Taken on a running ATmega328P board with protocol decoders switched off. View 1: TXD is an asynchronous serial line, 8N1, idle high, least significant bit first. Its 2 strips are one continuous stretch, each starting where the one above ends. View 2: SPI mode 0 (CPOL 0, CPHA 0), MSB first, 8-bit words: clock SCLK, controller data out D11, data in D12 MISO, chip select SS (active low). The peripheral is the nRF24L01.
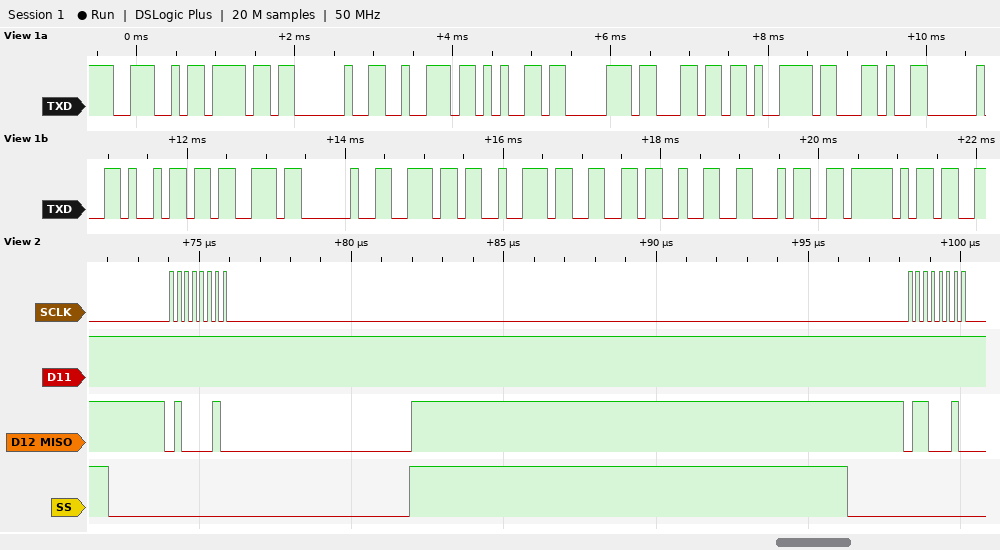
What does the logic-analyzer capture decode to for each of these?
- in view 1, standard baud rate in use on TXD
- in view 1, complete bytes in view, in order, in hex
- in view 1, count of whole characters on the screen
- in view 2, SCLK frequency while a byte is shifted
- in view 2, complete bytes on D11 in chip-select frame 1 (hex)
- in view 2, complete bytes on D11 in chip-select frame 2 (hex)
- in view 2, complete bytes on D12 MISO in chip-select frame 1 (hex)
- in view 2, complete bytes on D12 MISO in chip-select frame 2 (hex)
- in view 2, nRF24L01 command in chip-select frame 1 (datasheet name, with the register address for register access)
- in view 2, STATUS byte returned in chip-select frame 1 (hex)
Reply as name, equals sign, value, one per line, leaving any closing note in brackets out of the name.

in view 1, standard baud rate in use on TXD = 9600 baud
in view 1, complete bytes in view, in order, in hex = 0x4E 0x6F 0x20 0x72 0x65 0x70 0x6C 0x79 0x2C 0x20 0x69 0x73 0x20 0x6E 0x72 0x66 0x32 0x34 0x5F
in view 1, count of whole characters on the screen = 19
in view 2, SCLK frequency while a byte is shifted = 4 MHz
in view 2, complete bytes on D11 in chip-select frame 1 = FF
in view 2, complete bytes on D11 in chip-select frame 2 = FF
in view 2, complete bytes on D12 MISO in chip-select frame 1 = 42
in view 2, complete bytes on D12 MISO in chip-select frame 2 = 62
in view 2, nRF24L01 command in chip-select frame 1 = NOP
in view 2, STATUS byte returned in chip-select frame 1 = 0x42
